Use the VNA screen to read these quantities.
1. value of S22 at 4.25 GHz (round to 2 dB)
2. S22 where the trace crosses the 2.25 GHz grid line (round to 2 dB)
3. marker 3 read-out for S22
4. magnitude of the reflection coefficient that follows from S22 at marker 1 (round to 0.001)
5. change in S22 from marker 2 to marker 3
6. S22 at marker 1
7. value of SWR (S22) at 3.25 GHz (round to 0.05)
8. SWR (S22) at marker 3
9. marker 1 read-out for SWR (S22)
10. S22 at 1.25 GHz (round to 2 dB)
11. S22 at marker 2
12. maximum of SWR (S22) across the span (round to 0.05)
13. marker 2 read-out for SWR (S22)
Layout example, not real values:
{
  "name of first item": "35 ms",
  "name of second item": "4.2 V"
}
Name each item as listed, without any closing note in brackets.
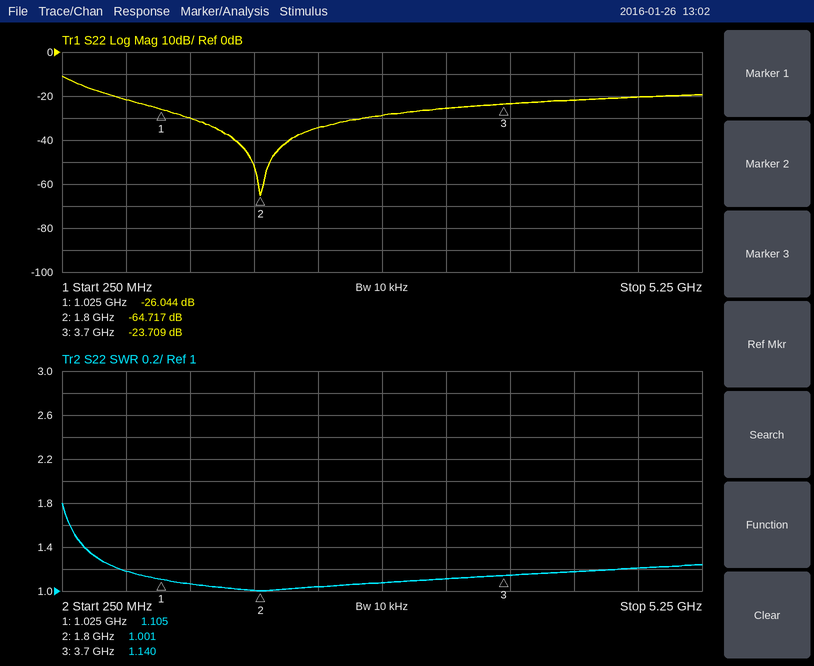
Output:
{
  "value of S22 at 4.25 GHz": "-22 dB",
  "S22 where the trace crosses the 2.25 GHz grid line": "-34 dB",
  "marker 3 read-out for S22": "-23.709 dB",
  "magnitude of the reflection coefficient that follows from S22 at marker 1": "0.050",
  "change in S22 from marker 2 to marker 3": "41.008 dB",
  "S22 at marker 1": "-26.044 dB",
  "value of SWR (S22) at 3.25 GHz": "1.10",
  "SWR (S22) at marker 3": "1.140",
  "marker 1 read-out for SWR": "1.105",
  "S22 at 1.25 GHz": "-30 dB",
  "S22 at marker 2": "-64.717 dB",
  "maximum of SWR (S22) across the span": "1.80",
  "marker 2 read-out for SWR": "1.001"
}
